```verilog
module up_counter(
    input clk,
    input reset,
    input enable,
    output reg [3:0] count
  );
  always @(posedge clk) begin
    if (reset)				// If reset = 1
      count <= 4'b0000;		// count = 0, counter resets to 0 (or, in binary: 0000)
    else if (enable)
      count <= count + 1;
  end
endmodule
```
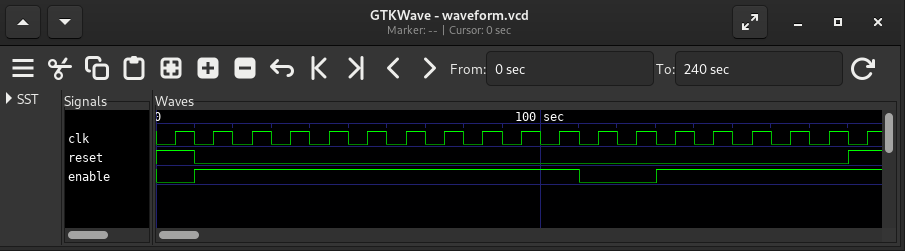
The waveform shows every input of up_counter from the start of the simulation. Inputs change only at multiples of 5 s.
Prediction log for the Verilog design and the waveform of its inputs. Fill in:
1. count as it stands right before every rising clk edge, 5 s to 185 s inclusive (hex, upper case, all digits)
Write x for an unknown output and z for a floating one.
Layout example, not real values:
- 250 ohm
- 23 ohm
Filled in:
- x, 0, 1, 2, 3, 4, 5, 6, 7, 8, 9, A, A, A, B, C, D, E, F
